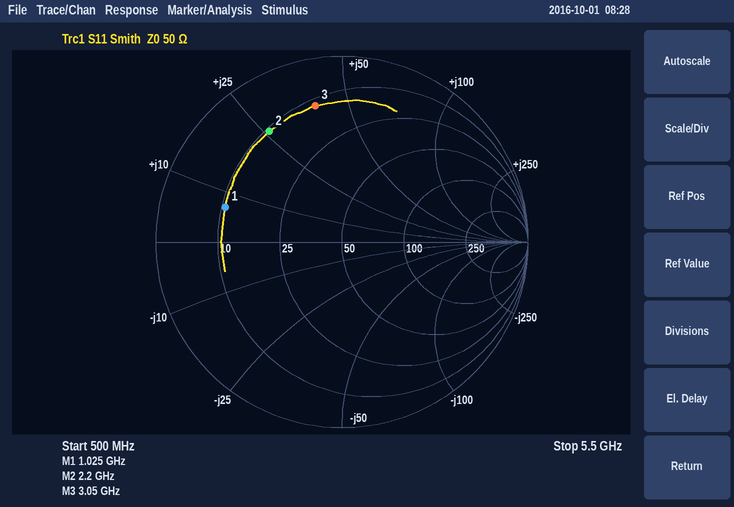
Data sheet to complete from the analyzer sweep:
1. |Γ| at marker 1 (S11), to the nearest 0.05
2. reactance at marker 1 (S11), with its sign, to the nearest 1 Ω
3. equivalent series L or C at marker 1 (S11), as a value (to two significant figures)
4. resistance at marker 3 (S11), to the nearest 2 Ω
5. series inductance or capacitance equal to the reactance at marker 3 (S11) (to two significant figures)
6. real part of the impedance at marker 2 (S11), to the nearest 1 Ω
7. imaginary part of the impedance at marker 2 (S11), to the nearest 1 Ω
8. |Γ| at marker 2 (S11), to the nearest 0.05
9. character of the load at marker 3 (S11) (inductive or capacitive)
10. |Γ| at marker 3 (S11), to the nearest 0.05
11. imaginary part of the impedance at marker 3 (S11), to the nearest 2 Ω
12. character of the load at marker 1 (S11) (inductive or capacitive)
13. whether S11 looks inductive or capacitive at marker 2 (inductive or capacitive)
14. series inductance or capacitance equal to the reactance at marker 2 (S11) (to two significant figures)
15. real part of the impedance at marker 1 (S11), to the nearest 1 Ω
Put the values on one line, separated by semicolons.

0.65; +7 Ω; 1.1 nH; 12 Ω; 2.1 nH; 11 Ω; +26 Ω; 0.70; inductive; 0.75; +40 Ω; inductive; inductive; 1.9 nH; 11 Ω
